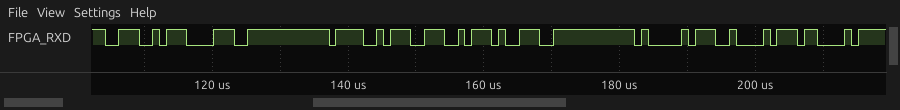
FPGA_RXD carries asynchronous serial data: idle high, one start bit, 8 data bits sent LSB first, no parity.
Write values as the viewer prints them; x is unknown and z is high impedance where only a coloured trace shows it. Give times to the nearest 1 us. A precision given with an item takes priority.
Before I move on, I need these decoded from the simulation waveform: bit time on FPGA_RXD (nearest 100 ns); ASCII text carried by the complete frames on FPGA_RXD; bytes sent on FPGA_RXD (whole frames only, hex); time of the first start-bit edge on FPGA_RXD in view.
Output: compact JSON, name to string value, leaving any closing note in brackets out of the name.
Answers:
{"bit time on FPGA_RXD": "1000 ns", "ASCII text carried by the complete frames on FPGA_RXD": "\"N8ON9ABC\"", "bytes sent on FPGA_RXD": "4E, 38, 4F, 4E, 39, 41, 42, 43", "time of the first start-bit edge on FPGA_RXD in view": "104 us"}
